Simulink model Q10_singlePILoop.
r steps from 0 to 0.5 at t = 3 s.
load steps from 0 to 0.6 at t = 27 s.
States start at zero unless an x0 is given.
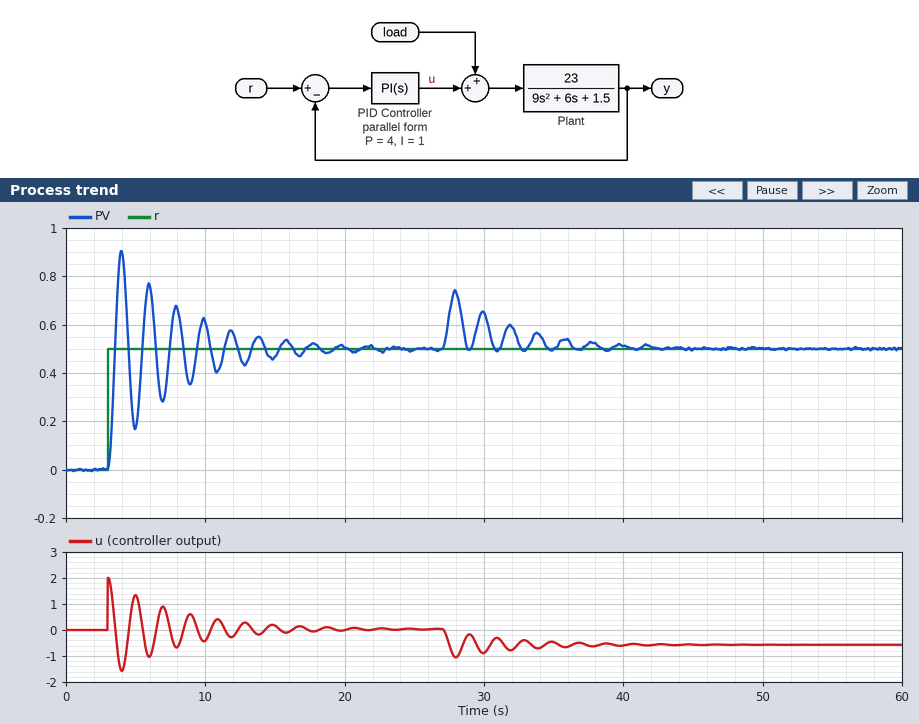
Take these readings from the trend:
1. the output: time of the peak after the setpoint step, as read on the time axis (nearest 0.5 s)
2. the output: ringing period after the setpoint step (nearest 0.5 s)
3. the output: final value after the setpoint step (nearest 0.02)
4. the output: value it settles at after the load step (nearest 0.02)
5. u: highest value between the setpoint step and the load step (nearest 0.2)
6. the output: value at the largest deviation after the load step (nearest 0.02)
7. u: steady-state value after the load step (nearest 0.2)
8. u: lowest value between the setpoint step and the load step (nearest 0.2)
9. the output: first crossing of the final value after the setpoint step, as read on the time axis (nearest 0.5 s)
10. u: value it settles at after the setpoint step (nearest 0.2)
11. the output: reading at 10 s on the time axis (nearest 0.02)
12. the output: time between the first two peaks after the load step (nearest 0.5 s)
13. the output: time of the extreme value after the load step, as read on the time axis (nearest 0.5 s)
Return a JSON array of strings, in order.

["4.0 s", "2.0 s", "0.50", "0.50", "2.0", "0.74", "-0.6", "-1.6", "3.5 s", "0.0", "0.60", "2.0 s", "28.0 s"]
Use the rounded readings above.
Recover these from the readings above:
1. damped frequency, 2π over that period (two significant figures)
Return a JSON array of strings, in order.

["3.1 rad/s"]
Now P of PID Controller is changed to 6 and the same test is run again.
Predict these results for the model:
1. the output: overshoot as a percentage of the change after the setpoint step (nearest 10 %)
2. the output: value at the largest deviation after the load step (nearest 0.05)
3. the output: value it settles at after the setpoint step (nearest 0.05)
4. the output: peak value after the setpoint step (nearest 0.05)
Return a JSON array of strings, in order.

["80 %", "0.65", "0.50", "0.90"]
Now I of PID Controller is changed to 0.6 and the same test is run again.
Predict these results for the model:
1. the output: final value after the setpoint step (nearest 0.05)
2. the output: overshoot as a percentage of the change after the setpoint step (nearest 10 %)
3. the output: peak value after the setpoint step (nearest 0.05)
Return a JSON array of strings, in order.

["0.50", "80 %", "0.90"]
